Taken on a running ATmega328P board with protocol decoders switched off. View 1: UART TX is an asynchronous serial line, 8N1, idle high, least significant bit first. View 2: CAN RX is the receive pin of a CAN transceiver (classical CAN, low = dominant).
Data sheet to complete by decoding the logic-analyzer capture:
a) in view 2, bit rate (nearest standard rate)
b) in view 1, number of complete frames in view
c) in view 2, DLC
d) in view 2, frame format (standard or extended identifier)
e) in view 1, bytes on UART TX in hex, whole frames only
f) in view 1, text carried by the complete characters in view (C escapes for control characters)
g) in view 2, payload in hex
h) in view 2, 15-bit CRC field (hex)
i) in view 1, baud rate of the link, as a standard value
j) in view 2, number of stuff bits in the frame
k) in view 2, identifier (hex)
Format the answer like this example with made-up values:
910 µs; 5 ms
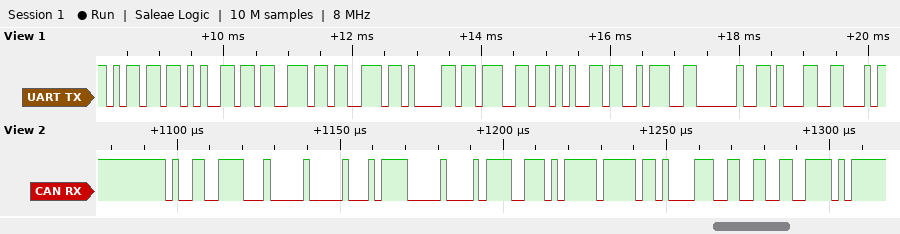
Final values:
500 kbit/s; 10; 8; standard; 6D 65 73 73 61 67 65 3A 20 31; "message: 1"; 00 2F 00 5E 75 FF E8 73; 0x199E; 9600 baud; 5; 0x4CF
